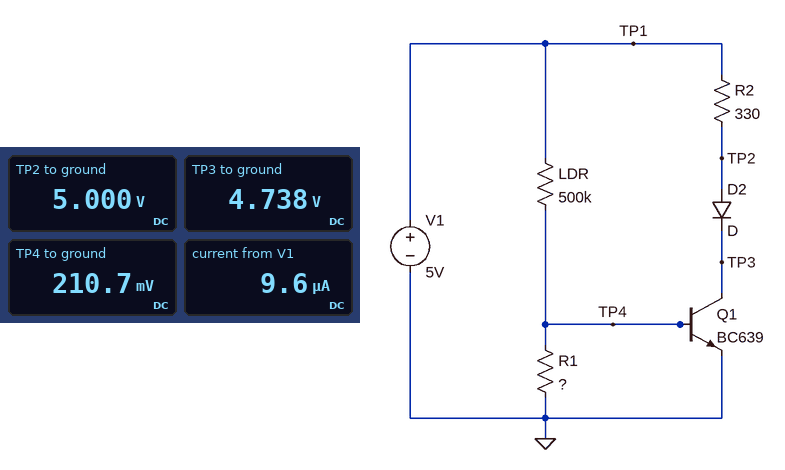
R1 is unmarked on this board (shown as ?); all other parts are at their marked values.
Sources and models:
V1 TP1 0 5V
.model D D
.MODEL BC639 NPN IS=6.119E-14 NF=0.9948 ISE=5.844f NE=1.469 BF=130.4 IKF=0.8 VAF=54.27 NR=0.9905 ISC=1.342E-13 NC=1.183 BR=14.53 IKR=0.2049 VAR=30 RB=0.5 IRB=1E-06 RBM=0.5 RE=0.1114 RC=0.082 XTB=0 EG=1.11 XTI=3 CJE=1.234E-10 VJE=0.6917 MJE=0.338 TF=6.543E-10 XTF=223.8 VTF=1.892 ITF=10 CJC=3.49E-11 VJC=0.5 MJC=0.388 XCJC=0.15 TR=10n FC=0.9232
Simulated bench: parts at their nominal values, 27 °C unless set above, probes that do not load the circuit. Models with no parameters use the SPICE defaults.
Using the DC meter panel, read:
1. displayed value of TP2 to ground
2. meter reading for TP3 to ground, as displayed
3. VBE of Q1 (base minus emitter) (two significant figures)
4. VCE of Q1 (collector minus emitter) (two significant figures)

5.000 V
4.738 V
210 mV
4.7 V
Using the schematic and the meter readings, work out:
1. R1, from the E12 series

22 kΩ
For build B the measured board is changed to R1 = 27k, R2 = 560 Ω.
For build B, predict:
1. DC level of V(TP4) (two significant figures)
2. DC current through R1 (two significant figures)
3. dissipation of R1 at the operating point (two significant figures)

260 mV
9.5 µA
2.4 µW
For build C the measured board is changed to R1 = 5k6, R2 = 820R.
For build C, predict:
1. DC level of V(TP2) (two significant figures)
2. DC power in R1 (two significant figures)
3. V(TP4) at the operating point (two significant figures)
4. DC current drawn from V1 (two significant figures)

5.0 V
550 nW
55 mV
9.9 µA
